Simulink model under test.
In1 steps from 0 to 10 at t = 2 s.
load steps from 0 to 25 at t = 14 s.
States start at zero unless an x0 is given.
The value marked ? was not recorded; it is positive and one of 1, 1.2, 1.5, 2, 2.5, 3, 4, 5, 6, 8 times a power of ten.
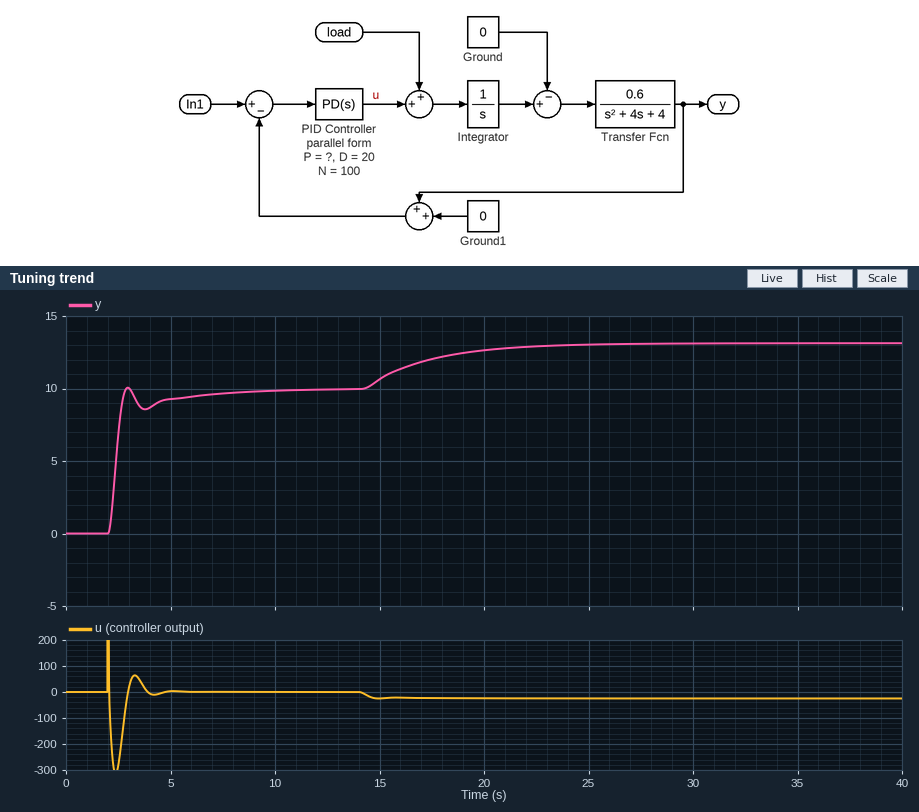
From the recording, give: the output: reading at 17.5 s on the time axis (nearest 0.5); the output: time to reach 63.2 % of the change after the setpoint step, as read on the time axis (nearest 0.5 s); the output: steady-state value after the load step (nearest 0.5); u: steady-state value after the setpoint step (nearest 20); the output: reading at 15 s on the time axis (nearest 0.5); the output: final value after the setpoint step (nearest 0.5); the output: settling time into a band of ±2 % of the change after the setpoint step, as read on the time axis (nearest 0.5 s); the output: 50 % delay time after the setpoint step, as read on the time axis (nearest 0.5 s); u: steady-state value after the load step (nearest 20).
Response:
12.0
2.5 s
13.0
0
10.5
10.0
9.0 s
2.5 s
-20
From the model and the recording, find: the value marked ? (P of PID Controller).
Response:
8
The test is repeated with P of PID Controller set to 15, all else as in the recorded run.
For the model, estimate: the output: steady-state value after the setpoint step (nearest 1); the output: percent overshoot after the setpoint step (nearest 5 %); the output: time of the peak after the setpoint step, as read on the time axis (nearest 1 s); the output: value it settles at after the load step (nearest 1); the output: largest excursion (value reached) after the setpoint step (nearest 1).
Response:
10
10 %
3 s
12
11
